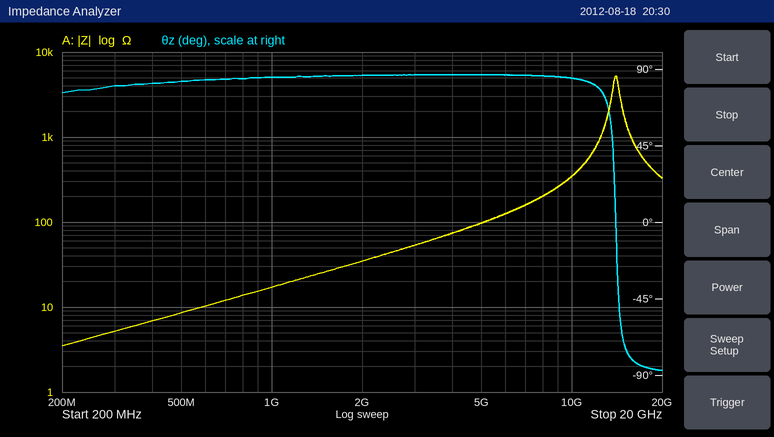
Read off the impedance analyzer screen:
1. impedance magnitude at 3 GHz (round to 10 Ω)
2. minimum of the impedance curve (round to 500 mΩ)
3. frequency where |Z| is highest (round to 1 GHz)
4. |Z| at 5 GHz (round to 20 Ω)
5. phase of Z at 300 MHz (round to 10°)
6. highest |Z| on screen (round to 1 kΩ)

50 Ω
3.5 Ω
14 GHz
100 Ω
80°
5 kΩ
